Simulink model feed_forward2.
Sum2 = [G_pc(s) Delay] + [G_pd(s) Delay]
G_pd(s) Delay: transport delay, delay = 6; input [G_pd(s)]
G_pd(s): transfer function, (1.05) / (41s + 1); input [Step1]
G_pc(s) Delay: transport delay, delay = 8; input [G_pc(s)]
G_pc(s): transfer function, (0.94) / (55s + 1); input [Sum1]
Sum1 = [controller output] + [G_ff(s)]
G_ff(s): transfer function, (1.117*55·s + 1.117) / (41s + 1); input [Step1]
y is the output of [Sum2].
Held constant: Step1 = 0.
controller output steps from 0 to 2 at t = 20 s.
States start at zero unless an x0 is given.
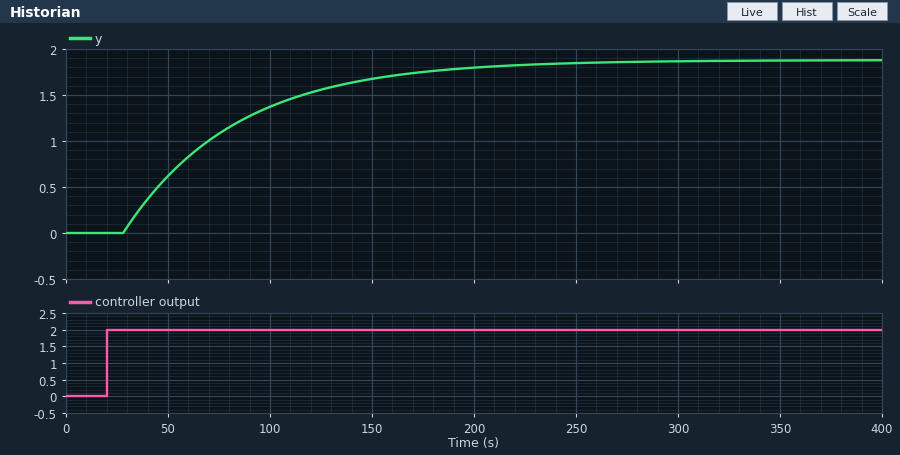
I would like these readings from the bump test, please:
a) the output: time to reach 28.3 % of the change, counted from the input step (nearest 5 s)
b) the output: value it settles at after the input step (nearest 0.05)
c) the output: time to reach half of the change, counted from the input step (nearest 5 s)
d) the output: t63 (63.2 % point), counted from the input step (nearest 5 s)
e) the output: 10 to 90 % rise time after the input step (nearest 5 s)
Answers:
25 s
1.90
45 s
65 s
120 s
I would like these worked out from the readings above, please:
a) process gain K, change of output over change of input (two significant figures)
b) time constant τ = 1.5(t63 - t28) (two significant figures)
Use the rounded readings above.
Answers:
0.95
60 s
